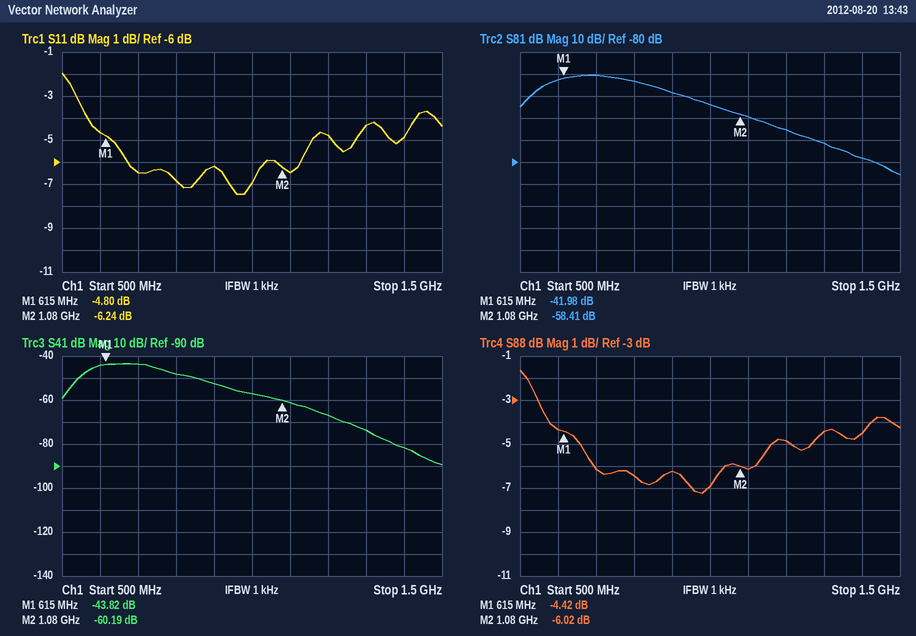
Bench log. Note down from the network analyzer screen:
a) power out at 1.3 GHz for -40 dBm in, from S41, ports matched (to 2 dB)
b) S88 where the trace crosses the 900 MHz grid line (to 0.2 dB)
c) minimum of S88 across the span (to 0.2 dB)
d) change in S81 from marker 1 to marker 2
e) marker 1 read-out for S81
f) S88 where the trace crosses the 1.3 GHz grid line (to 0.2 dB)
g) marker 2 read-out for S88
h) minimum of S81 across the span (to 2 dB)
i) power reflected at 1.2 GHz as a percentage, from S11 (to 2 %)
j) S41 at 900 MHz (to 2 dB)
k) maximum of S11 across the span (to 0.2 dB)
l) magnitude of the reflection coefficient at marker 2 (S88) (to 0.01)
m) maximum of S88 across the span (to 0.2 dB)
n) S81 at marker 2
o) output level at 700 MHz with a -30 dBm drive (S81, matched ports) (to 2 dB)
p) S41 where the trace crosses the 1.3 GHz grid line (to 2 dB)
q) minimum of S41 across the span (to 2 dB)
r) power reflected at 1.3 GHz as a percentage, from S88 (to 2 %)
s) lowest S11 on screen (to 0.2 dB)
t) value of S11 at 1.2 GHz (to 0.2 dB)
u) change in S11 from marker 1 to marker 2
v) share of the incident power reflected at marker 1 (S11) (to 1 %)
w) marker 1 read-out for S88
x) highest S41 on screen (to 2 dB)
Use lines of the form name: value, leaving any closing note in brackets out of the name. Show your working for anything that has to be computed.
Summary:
power out at 1.3 GHz for -40 dBm in, from S41, ports matched: -40 dBm + (-74 dB) = -114 dBm
S88 where the trace crosses the 900 MHz grid line: -6.2 dB
minimum of S88 across the span: -7.2 dB
change in S81 from marker 1 to marker 2: -58.41 − (-41.98) = -16.43 dB
marker 1 read-out for S81: -41.98 dB
S88 where the trace crosses the 1.3 GHz grid line: -4.4 dB
marker 2 read-out for S88: -6.02 dB
minimum of S81 across the span: -86 dB
power reflected at 1.2 GHz as a percentage, from S11: 10^(-4.8/10) ≈ 33.1 %, so 34 % to the nearest 2 %
S41 at 900 MHz: -52 dB
maximum of S11 across the span: -2.0 dB
magnitude of the reflection coefficient at marker 2 (S88): 10^(-6.02/20) ≈ 0.50
maximum of S88 across the span: -1.6 dB
S81 at marker 2: -58.41 dB
output level at 700 MHz with a -30 dBm drive (S81, matched ports): -30 dBm + (-40 dB) = -70 dBm
S41 where the trace crosses the 1.3 GHz grid line: -74 dB
minimum of S41 across the span: -90 dB
power reflected at 1.3 GHz as a percentage, from S88: 10^(-4.4/10) ≈ 36 %
lowest S11 on screen: -7.4 dB
value of S11 at 1.2 GHz: -4.8 dB
change in S11 from marker 1 to marker 2: -6.24 − (-4.8) = -1.44 dB
share of the incident power reflected at marker 1 (S11): 10^(-4.8/10) ≈ 33 %
marker 1 read-out for S88: -4.42 dB
highest S41 on screen: -44 dB
